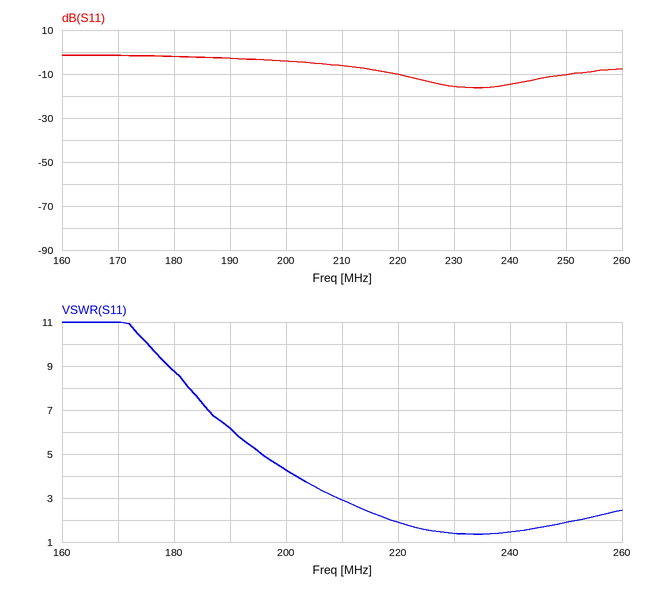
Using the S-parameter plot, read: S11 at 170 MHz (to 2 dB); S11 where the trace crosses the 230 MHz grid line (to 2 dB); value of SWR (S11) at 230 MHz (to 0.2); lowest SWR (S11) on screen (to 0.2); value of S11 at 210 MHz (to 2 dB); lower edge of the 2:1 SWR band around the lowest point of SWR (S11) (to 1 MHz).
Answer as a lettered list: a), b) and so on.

a) -2 dB
b) -16 dB
c) 1.4
d) 1.4
e) -6 dB
f) 219 MHz
